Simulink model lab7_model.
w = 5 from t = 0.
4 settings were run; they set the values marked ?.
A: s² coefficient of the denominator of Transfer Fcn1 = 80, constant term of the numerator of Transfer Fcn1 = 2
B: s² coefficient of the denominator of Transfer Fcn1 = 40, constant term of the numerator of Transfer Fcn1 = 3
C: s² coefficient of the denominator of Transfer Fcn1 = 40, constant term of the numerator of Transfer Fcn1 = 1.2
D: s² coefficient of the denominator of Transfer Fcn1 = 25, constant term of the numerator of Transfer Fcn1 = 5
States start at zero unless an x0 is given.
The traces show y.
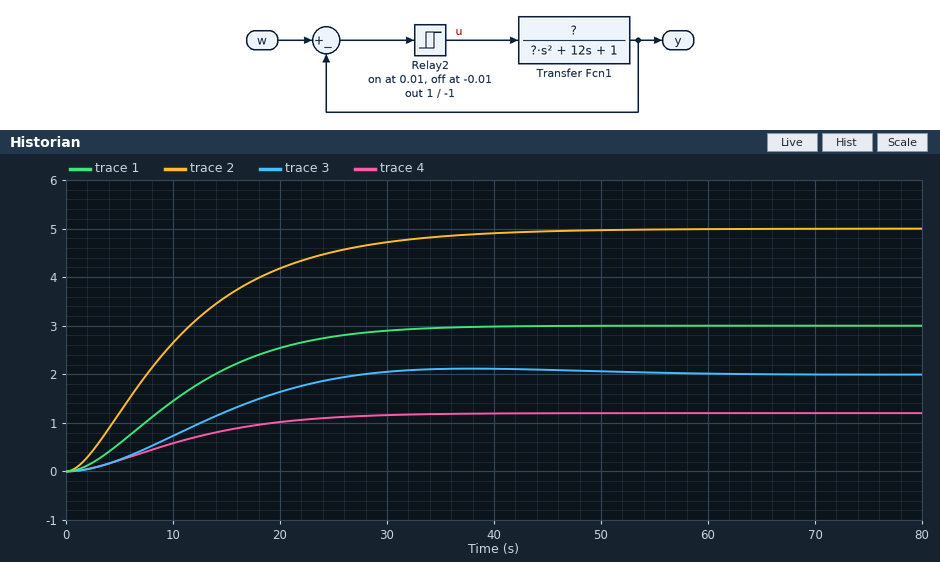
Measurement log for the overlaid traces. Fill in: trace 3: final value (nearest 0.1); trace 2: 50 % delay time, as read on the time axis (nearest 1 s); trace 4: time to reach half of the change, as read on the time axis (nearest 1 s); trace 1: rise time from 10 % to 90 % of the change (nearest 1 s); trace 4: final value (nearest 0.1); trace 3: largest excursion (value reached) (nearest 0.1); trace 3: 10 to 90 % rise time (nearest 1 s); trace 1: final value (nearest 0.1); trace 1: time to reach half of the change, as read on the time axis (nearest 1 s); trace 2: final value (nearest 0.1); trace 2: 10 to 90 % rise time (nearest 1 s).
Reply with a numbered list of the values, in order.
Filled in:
1. 2.0
2. 9 s
3. 10 s
4. 20 s
5. 1.2
6. 2.1
7. 18 s
8. 3.0
9. 10 s
10. 5.0
11. 22 s
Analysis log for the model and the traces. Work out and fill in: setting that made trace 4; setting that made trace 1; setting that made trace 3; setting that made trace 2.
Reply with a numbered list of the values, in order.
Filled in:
1. C
2. B
3. A
4. D
